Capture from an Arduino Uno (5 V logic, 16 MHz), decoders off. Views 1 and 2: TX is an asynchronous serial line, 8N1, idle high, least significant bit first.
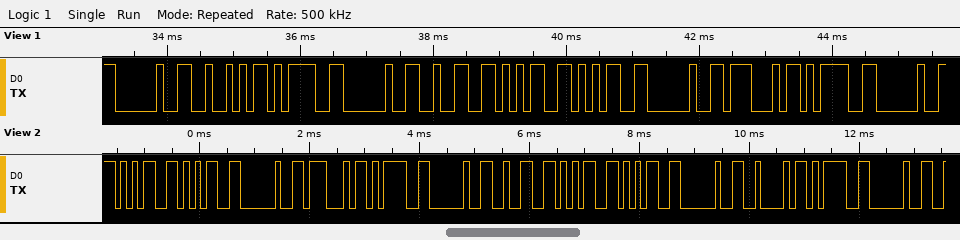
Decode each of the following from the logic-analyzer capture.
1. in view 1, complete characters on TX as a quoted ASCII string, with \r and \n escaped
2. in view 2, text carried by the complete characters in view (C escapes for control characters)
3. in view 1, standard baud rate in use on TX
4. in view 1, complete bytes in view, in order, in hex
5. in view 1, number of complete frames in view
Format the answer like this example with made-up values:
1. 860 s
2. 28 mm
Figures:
1. " R= 255 G= "
2. "55 G= 255 B= "
3. 9600 baud
4. 0x20 0x52 0x3D 0x20 0x32 0x35 0x35 0x20 0x47 0x3D 0x20
5. 11
